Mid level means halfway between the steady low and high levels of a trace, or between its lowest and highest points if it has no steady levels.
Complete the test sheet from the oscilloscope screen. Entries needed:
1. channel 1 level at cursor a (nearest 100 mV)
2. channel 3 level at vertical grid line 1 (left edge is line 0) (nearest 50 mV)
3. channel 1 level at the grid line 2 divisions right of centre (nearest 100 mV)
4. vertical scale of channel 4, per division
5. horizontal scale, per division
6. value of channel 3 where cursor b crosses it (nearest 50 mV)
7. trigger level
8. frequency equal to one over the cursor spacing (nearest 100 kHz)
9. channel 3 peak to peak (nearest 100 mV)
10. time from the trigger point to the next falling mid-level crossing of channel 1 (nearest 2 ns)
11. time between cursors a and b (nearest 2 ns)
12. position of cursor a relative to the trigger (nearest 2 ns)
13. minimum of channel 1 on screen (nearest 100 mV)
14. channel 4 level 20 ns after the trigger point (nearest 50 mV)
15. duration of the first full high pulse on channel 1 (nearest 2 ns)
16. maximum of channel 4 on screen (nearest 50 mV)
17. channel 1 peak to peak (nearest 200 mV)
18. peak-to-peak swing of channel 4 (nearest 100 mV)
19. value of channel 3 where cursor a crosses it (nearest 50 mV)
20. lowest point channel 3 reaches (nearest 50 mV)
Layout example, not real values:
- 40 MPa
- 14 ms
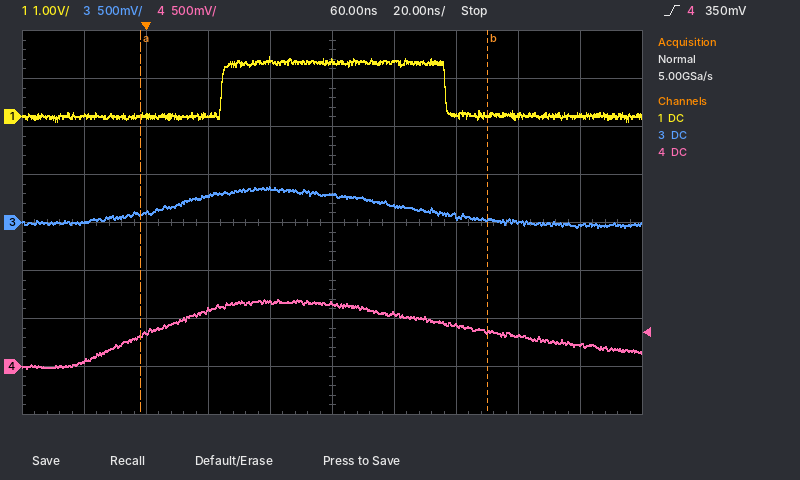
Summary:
- 0.0 V
- 0 mV
- 0.0 V
- 500 mV
- 20 ns
- 50 mV
- 350 mV
- 8.9 MHz
- 400 mV
- 96 ns
- 112 ns
- -2 ns
- -100 mV
- 600 mV
- 72 ns
- 700 mV
- 1.4 V
- 700 mV
- 100 mV
- -50 mV
